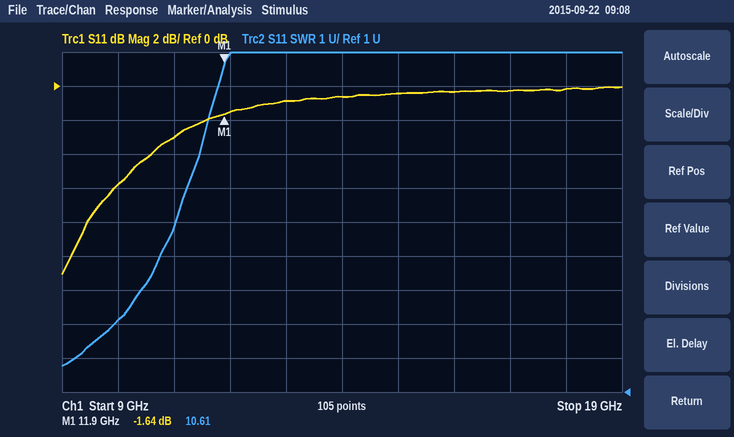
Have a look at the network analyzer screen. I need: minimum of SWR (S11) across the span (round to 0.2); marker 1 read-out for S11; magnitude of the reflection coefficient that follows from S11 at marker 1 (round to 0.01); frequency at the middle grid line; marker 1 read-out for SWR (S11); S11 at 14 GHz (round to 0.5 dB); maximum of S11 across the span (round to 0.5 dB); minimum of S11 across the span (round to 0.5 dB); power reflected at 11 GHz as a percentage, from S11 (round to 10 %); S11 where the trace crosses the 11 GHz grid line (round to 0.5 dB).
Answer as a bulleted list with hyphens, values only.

- 1.8
- -1.64 dB
- 0.83
- 14 GHz
- 10.61
- -0.5 dB
- 0.0 dB
- -11.0 dB
- 50 %
- -3.0 dB
